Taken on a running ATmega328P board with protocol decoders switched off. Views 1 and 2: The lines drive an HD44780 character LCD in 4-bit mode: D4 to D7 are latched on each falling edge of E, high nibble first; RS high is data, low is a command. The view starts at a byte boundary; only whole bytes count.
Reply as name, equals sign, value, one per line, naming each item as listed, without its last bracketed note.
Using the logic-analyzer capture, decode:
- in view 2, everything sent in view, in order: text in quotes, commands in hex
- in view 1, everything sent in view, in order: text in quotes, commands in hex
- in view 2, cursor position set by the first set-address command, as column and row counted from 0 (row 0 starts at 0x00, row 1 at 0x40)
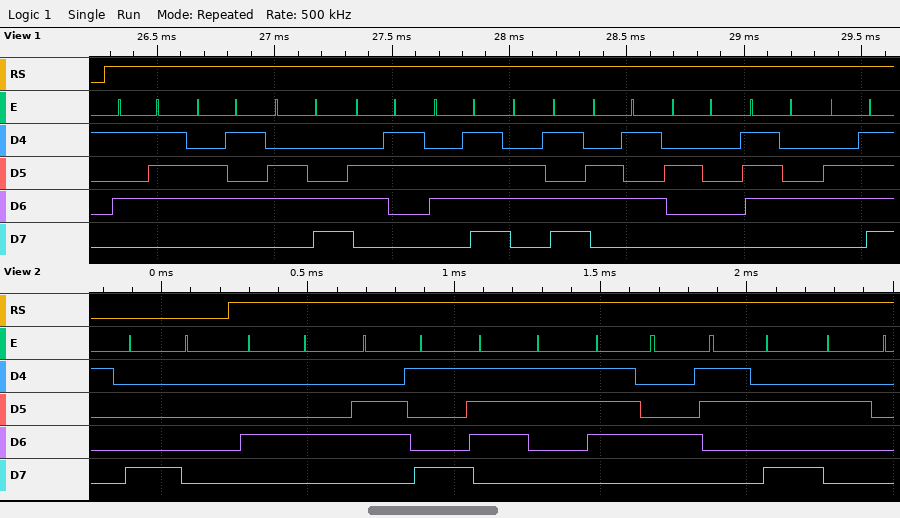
in view 2, everything sent in view, in order: text in quotes, commands in hex = 0x80 "Dist: "
in view 1, everything sent in view, in order: text in quotes, commands in hex = "Welcome to"
in view 2, cursor position set by the first set-address command, as column and row counted from 0 = column 0, row 0
